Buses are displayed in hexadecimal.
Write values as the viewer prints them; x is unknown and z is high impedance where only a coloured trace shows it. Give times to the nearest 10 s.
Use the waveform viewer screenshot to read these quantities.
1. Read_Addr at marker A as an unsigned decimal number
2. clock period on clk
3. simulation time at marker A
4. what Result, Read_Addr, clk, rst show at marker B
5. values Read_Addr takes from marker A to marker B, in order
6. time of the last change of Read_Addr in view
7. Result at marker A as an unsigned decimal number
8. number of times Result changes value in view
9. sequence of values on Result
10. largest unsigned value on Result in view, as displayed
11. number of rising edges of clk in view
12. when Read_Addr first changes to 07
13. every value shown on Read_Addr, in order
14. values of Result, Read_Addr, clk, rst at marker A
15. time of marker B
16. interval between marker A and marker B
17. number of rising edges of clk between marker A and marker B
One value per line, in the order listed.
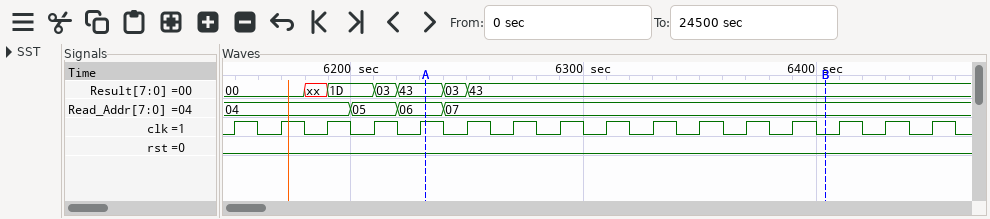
6
20 s
6230 s
Result=43, Read_Addr=07, clk=0, rst=0
06, 07
6240 s
67
6
00, xx, 1D, 03, 43, 03, 43
43
16
6240 s
04, 05, 06, 07
Result=43, Read_Addr=06, clk=1, rst=0
6400 s
170 s
8
